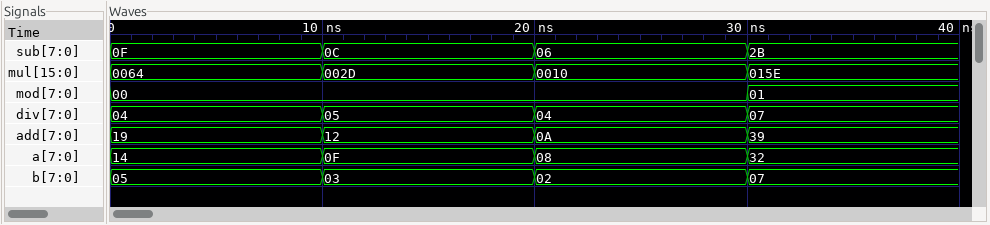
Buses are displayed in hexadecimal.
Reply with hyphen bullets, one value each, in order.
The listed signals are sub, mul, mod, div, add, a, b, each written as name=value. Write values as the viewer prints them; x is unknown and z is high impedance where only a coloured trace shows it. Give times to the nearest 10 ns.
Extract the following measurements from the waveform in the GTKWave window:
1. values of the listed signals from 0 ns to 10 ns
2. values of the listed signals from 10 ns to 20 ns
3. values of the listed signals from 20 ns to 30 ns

- sub=0F, mul=0064, mod=00, div=04, add=19, a=14, b=05
- sub=0C, mul=002D, mod=00, div=05, add=12, a=0F, b=03
- sub=06, mul=0010, mod=00, div=04, add=0A, a=08, b=02
